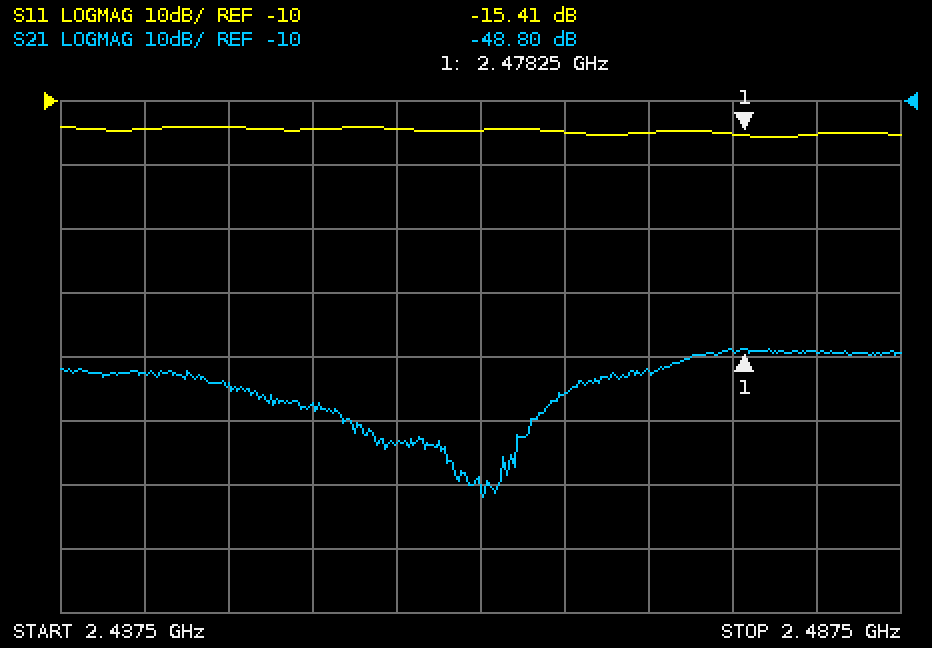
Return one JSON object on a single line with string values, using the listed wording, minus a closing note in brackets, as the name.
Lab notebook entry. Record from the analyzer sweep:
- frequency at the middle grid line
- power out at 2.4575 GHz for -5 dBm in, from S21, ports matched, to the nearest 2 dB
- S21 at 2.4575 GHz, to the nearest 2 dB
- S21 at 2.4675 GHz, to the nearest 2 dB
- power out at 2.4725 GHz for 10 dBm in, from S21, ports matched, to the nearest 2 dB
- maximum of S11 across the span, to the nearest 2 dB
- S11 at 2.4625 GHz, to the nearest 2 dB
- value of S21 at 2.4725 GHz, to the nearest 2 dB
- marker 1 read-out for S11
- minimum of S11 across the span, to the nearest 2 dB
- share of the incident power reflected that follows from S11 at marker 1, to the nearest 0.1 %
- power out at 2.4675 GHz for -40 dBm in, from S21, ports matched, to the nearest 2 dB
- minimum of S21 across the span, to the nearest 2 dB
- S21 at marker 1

{"frequency at the middle grid line": "2.4625 GHz", "power out at 2.4575 GHz for -5 dBm in, from S21, ports matched, to the nearest 2 dB": "-68 dBm", "S21 at 2.4575 GHz, to the nearest 2 dB": "-64 dB", "S21 at 2.4675 GHz, to the nearest 2 dB": "-56 dB", "power out at 2.4725 GHz for 10 dBm in, from S21, ports matched, to the nearest 2 dB": "-42 dBm", "maximum of S11 across the span, to the nearest 2 dB": "-14 dB", "S11 at 2.4625 GHz, to the nearest 2 dB": "-14 dB", "value of S21 at 2.4725 GHz, to the nearest 2 dB": "-52 dB", "marker 1 read-out for S11": "-15.41 dB", "minimum of S11 across the span, to the nearest 2 dB": "-16 dB", "share of the incident power reflected that follows from S11 at marker 1, to the nearest 0.1 %": "2.9 %", "power out at 2.4675 GHz for -40 dBm in, from S21, ports matched, to the nearest 2 dB": "-96 dBm", "minimum of S21 across the span, to the nearest 2 dB": "-72 dB", "S21 at marker 1": "-48.80 dB"}
